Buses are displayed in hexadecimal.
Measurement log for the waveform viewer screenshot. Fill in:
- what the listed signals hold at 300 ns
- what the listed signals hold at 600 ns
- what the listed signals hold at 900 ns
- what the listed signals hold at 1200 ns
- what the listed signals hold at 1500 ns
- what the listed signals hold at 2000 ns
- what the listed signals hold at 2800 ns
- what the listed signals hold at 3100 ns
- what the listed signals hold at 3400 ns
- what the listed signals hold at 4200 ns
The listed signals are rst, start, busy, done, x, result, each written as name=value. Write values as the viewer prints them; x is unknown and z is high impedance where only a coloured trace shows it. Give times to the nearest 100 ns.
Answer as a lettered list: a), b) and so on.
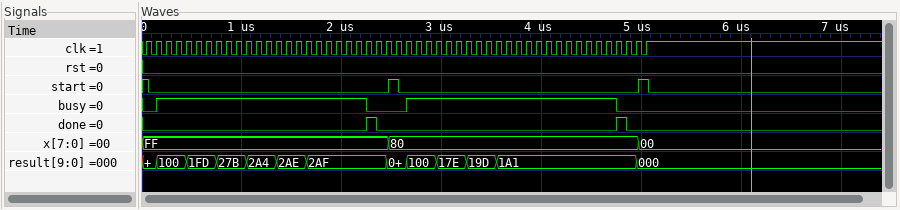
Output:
a) rst=0, start=0, busy=1, done=0, x=FF, result=100
b) rst=0, start=0, busy=1, done=0, x=FF, result=1FD
c) rst=0, start=0, busy=1, done=0, x=FF, result=27B
d) rst=0, start=0, busy=1, done=0, x=FF, result=2A4
e) rst=0, start=0, busy=1, done=0, x=FF, result=2AE
f) rst=0, start=0, busy=1, done=0, x=FF, result=2AF
g) rst=0, start=0, busy=1, done=0, x=80, result=100
h) rst=0, start=0, busy=1, done=0, x=80, result=17E
i) rst=0, start=0, busy=1, done=0, x=80, result=19D
j) rst=0, start=0, busy=1, done=0, x=80, result=1A1
